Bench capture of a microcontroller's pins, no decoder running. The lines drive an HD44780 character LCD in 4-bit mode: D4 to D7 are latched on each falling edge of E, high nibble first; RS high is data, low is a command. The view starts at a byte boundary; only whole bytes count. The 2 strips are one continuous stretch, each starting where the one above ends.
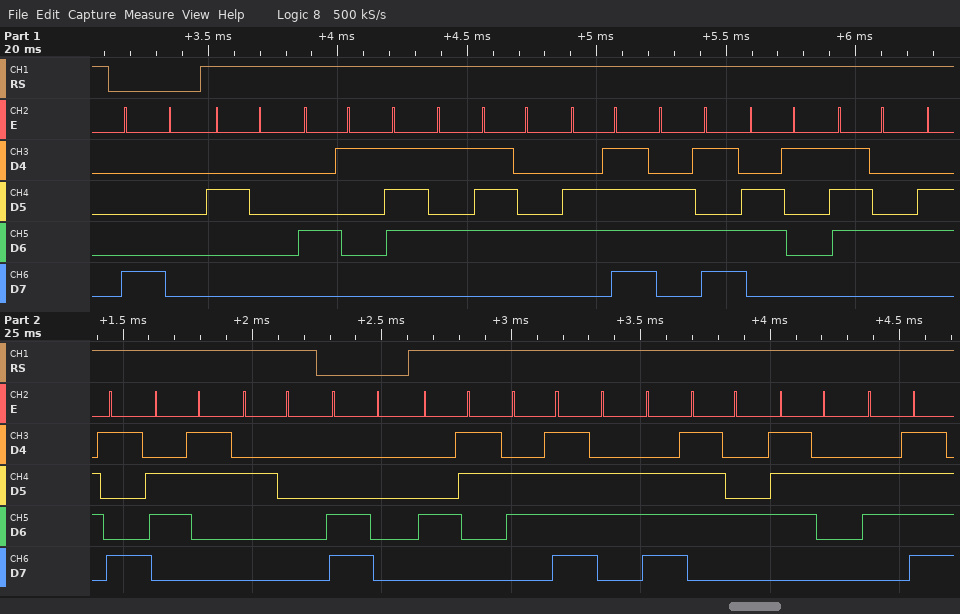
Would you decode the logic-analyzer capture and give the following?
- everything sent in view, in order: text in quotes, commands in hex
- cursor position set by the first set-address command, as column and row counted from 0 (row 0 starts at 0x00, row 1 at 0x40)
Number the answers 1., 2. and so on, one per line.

1. 0x80 " Automatic " 0xC0 "Contro"
2. column 0, row 0
